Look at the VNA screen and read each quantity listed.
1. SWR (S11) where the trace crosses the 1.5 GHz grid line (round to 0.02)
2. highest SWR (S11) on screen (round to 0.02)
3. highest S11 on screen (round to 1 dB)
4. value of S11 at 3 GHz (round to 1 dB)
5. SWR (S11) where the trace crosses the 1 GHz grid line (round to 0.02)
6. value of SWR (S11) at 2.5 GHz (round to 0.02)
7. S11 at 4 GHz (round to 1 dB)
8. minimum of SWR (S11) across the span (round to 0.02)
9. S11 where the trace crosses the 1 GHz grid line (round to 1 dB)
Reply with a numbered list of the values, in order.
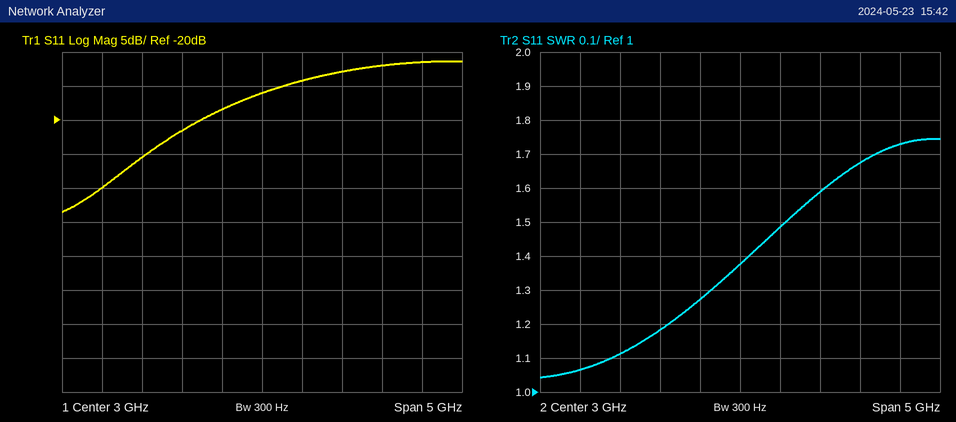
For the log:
1. 1.12
2. 1.74
3. -11 dB
4. -16 dB
5. 1.06
6. 1.28
7. -13 dB
8. 1.04
9. -30 dB
